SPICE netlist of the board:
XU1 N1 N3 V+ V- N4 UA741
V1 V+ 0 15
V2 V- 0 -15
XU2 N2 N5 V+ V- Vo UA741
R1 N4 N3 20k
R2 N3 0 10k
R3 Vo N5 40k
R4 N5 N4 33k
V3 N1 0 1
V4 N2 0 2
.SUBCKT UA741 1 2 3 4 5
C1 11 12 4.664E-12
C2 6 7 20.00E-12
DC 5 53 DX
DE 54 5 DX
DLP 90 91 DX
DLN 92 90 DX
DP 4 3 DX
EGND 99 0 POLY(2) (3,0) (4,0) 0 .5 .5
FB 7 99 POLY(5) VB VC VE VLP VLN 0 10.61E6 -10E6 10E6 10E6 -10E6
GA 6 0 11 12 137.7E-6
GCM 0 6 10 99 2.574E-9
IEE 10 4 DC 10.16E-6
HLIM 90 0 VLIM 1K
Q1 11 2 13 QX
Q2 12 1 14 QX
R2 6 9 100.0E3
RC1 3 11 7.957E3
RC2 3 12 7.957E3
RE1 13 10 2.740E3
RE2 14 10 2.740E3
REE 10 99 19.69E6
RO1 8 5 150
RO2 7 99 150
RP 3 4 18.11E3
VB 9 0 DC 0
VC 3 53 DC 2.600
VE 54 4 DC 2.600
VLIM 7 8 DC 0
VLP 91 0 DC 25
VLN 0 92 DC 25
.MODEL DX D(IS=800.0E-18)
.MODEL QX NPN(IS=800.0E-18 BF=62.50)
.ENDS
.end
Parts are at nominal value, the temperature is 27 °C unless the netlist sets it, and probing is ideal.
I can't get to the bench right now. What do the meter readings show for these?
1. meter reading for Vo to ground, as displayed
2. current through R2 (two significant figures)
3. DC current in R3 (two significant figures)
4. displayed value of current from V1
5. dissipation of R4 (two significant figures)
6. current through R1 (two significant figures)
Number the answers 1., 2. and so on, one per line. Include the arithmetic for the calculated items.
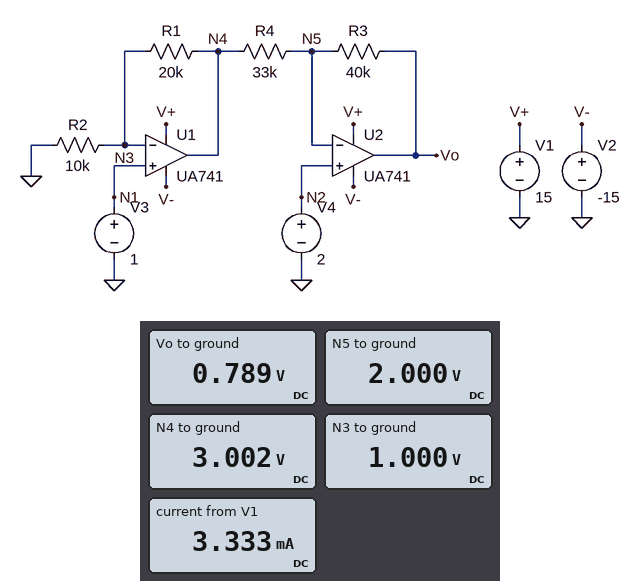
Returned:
1. 0.789 V
2. (1 V) / 10 kΩ = 100 µA
3. (2 V - 789 mV) / 40 kΩ = 30 µA
4. 3.333 mA
5. (3.002 V - 2 V)^2 / 33 kΩ = 30 µW
6. (3.002 V - 1 V) / 20 kΩ = 100 µA
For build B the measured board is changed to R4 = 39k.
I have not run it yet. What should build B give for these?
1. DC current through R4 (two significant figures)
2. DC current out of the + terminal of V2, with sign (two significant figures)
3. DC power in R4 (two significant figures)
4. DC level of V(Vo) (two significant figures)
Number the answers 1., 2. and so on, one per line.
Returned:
1. 26 µA
2. -3.3 mA
3. 26 µW
4. 980 mV
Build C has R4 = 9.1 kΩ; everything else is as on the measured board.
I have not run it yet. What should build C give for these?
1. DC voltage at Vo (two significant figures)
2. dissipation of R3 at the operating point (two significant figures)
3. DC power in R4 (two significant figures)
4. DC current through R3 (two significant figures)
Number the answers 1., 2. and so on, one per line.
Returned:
1. -2.4 V
2. 480 µW
3. 110 µW
4. 110 µA
